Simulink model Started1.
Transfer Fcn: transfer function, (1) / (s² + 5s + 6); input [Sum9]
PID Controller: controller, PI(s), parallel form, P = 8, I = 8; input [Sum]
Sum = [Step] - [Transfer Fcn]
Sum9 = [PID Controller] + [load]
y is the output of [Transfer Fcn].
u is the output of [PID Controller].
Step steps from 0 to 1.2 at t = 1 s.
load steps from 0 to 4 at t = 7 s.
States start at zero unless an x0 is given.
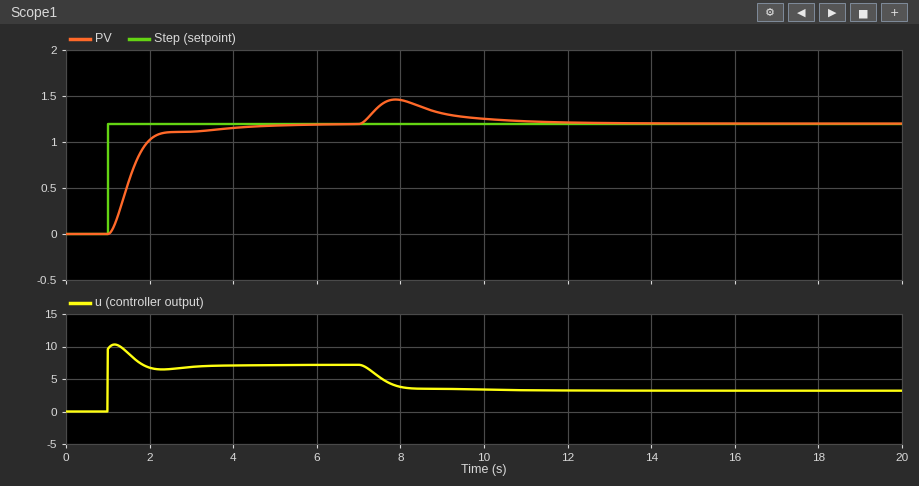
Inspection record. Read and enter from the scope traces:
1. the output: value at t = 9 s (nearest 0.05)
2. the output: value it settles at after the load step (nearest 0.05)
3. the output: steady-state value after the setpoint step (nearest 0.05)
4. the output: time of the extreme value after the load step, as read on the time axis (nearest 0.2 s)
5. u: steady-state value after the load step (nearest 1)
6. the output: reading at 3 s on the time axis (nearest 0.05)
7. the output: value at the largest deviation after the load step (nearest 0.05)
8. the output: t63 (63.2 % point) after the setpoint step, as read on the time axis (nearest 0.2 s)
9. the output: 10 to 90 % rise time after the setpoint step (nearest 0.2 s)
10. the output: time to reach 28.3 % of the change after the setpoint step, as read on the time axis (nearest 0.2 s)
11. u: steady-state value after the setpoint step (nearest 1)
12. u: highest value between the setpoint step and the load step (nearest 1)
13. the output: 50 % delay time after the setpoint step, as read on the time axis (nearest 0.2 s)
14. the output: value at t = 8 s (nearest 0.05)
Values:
1.30
1.20
1.20
7.8 s
3
1.10
1.45
1.6 s
1.0 s
1.4 s
7
10
1.6 s
1.45
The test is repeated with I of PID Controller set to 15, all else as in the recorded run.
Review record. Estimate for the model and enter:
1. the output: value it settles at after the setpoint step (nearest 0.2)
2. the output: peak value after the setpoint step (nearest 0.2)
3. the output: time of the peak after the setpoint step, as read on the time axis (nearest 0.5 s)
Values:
1.2
1.4
2.5 s
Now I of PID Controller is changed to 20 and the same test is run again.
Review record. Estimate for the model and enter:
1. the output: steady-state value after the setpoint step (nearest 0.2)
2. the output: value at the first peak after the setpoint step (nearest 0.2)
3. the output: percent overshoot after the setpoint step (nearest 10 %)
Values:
1.2
1.4
20 %
